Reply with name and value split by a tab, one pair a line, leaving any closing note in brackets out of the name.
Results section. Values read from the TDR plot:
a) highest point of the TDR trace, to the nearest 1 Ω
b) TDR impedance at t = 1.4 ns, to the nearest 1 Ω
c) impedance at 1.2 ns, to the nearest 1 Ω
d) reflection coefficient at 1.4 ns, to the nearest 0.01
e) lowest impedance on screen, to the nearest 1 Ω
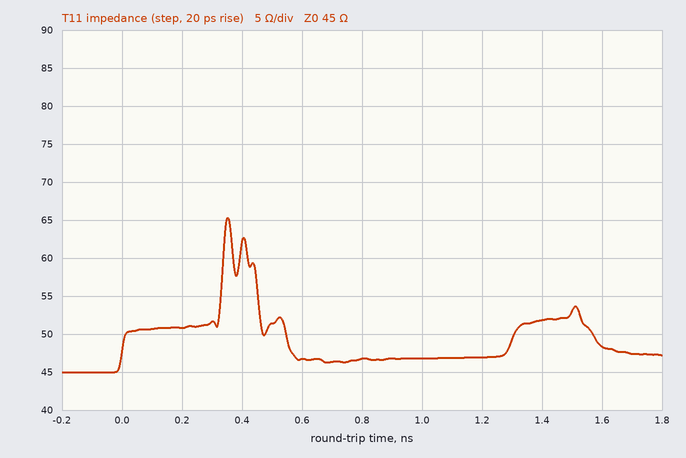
highest point of the TDR trace, to the nearest 1 Ω	65 Ω
TDR impedance at t = 1.4 ns, to the nearest 1 Ω	52 Ω
impedance at 1.2 ns, to the nearest 1 Ω	47 Ω
reflection coefficient at 1.4 ns, to the nearest 0.01	+0.07
lowest impedance on screen, to the nearest 1 Ω	45 Ω
